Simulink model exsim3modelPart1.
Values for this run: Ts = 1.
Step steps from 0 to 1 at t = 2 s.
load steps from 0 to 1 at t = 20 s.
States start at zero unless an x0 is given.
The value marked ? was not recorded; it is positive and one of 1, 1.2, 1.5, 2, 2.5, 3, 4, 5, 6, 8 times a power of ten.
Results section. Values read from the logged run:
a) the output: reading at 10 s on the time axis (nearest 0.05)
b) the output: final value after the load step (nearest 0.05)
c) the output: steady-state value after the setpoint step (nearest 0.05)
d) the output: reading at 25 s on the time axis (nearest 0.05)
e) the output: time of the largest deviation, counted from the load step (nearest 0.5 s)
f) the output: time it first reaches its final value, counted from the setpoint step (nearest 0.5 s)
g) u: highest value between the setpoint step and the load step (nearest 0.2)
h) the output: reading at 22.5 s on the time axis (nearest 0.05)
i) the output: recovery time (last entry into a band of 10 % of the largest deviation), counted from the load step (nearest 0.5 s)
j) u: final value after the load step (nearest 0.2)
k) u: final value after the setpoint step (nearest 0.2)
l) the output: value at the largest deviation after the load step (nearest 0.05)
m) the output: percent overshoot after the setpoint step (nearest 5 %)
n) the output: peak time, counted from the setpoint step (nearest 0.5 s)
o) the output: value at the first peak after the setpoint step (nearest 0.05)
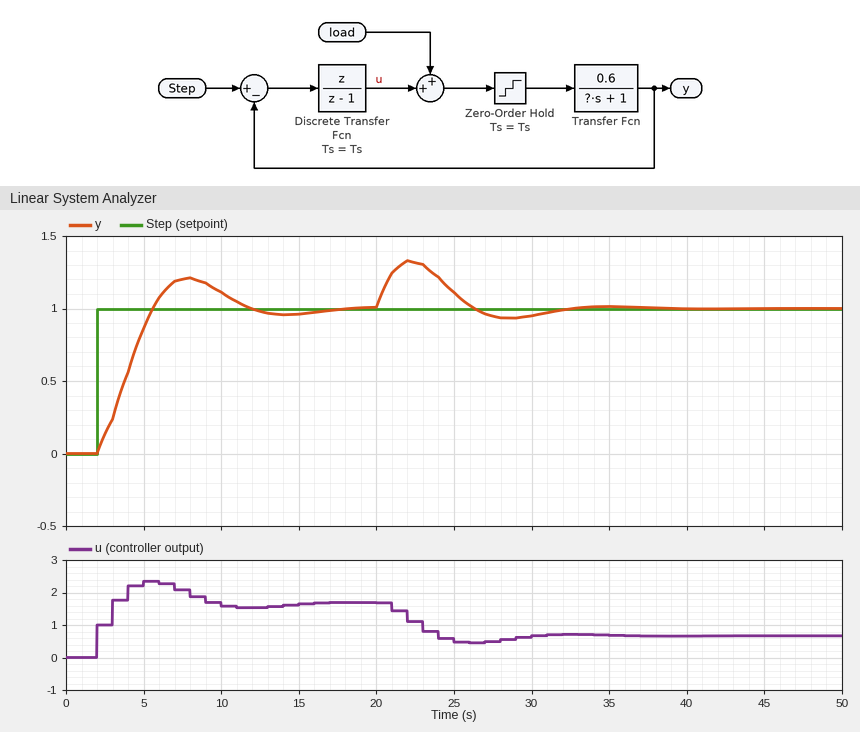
1.10
1.00
1.00
1.10
2.0 s
3.5 s
2.4
1.30
11.0 s
0.6
1.6
1.35
20 %
6.0 s
1.20
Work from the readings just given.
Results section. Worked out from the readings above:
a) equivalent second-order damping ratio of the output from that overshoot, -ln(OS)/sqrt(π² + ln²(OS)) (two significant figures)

0.46
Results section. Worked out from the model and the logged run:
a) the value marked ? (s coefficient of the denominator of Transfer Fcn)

2
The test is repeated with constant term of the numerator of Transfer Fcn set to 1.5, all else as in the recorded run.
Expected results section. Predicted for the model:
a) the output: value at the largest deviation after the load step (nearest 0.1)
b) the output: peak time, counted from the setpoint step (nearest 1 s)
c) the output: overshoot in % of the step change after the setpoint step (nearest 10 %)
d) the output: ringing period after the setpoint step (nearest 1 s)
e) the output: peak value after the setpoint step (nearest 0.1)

1.6
3 s
40 %
7 s
1.4
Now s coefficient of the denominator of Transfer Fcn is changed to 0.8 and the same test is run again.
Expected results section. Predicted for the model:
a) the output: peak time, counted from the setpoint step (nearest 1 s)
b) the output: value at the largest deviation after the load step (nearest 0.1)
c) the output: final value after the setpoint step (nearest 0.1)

4 s
1.4
1.0
